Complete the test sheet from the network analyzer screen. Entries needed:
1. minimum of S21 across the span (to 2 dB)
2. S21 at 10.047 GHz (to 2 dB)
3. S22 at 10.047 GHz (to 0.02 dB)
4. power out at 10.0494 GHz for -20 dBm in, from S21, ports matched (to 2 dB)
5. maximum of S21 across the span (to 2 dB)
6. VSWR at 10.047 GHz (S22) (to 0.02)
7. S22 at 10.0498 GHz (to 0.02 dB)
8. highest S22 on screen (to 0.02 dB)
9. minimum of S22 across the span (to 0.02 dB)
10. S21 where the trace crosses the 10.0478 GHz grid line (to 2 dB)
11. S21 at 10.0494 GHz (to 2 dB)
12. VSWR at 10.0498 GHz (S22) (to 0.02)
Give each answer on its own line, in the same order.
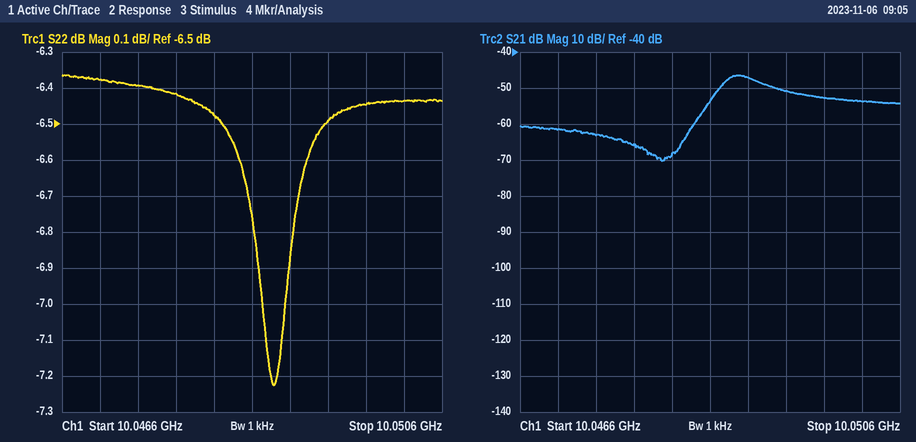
-70 dB
-62 dB
-6.38 dB
-70 dBm
-46 dB
2.84
-6.44 dB
-6.36 dB
-7.22 dB
-66 dB
-50 dB
2.82
